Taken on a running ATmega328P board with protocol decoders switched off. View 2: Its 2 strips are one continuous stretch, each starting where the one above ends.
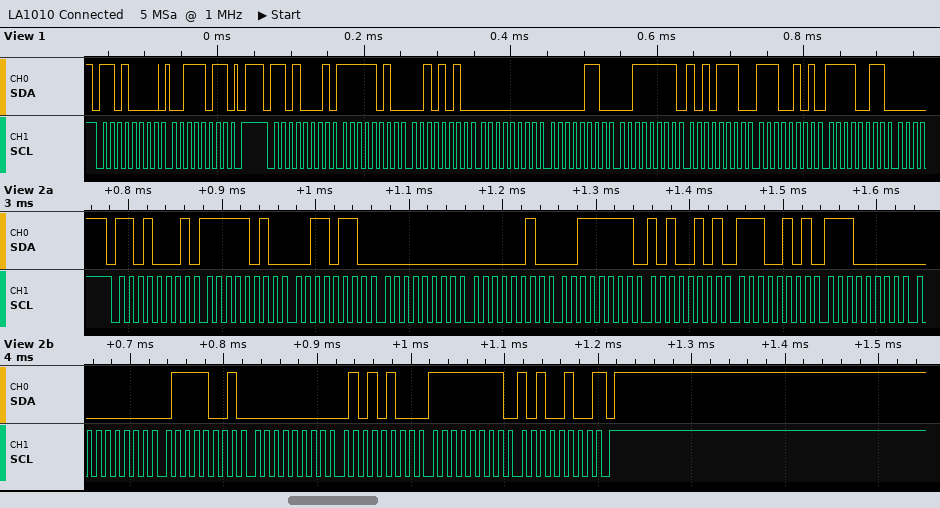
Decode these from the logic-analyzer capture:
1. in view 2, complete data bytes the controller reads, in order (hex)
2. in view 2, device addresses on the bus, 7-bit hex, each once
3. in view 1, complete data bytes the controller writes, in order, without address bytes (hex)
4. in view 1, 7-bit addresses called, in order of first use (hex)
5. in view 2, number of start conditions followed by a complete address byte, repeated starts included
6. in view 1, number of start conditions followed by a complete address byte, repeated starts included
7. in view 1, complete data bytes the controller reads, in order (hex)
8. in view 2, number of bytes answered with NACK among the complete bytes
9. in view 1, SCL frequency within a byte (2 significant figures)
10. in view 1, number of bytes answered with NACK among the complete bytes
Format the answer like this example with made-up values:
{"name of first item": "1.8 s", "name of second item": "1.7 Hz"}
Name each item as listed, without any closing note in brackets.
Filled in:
{"in view 2, complete data bytes the controller reads, in order": "FA 36 00 02 3F A5 E5 E0 00 79 00 54 FF A4", "in view 2, device addresses on the bus, 7-bit hex, each once": "0x68", "in view 1, complete data bytes the controller writes, in order, without address bytes": "3B", "in view 1, 7-bit addresses called, in order of first use": "0x68", "in view 2, number of start conditions followed by a complete address byte, repeated starts included": "1", "in view 1, number of start conditions followed by a complete address byte, repeated starts included": "2", "in view 1, complete data bytes the controller reads, in order": "FA 2A 00 06 3F AE E5 F3", "in view 2, number of bytes answered with NACK among the complete bytes": "1", "in view 1, SCL frequency within a byte": "100 kHz", "in view 1, number of bytes answered with NACK among the complete bytes": "0"}
